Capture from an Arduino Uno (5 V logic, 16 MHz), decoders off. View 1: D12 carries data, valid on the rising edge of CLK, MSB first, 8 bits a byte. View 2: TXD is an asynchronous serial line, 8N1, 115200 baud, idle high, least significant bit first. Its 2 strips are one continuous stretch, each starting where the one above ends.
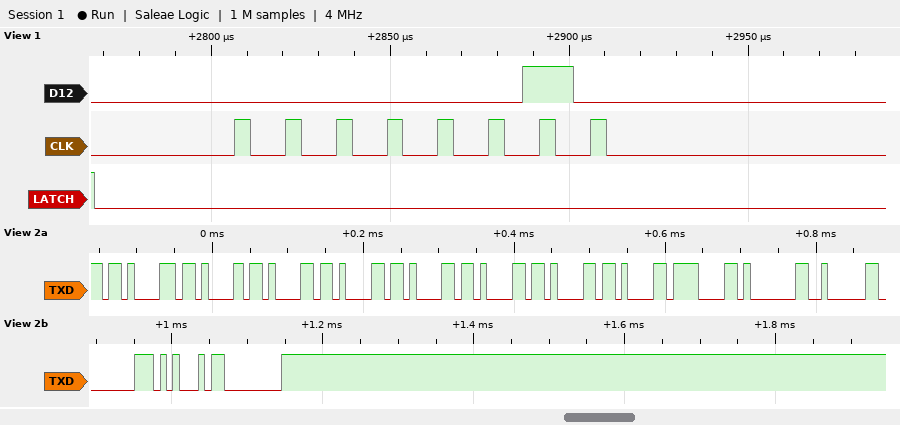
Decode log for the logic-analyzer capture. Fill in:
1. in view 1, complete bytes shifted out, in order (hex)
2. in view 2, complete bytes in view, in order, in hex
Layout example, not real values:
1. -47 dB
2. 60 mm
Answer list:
1. 02
2. 0x0B 0x0B 0x0B 0x0B 0x0B 0x0B 0x0B 0x0B 0x0F 0x01 0x02 0x80 0x45 0x00
